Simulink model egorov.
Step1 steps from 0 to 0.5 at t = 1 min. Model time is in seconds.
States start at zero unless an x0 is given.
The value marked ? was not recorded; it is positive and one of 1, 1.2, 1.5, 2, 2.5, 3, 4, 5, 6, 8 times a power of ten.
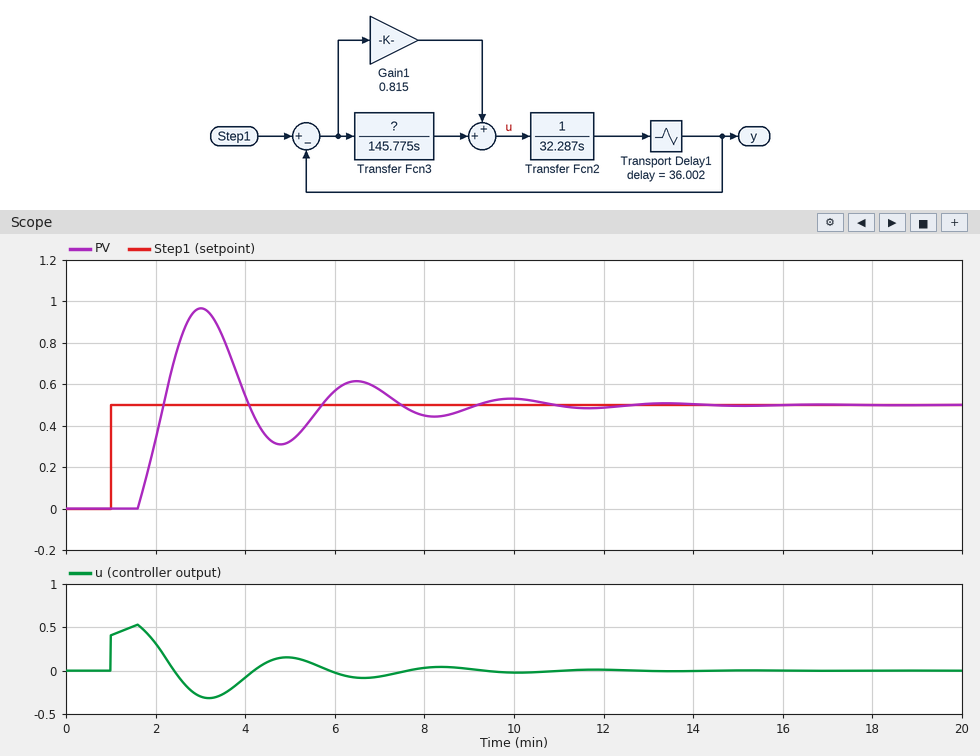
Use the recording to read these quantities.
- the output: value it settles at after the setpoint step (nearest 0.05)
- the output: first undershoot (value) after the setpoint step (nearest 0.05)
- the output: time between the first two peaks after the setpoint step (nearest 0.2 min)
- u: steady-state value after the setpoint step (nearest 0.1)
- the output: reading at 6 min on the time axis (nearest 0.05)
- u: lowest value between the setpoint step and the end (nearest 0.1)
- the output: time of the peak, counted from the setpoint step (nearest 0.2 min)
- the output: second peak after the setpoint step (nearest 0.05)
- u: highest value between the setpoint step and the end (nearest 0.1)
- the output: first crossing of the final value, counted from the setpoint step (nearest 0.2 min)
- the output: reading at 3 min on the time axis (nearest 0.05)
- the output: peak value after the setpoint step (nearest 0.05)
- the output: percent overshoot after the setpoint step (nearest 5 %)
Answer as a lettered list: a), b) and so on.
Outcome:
a) 0.50
b) 0.30
c) 3.4 min
d) 0.0
e) 0.55
f) -0.3
g) 2.0 min
h) 0.60
i) 0.5
j) 1.2 min
k) 0.95
l) 0.95
m) 95 %
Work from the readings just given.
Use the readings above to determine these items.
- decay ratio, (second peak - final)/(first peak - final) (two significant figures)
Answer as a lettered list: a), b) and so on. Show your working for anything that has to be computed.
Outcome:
a) (0.6 - 0.5) / (0.95 - 0.5) = 0.22
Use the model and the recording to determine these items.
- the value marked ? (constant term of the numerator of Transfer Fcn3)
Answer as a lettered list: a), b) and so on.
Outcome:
a) 1
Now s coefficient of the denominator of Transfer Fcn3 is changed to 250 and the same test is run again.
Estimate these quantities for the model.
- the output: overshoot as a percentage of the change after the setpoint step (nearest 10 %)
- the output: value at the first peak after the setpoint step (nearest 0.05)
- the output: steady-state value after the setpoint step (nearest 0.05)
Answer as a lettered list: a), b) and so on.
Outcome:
a) 70 %
b) 0.85
c) 0.50
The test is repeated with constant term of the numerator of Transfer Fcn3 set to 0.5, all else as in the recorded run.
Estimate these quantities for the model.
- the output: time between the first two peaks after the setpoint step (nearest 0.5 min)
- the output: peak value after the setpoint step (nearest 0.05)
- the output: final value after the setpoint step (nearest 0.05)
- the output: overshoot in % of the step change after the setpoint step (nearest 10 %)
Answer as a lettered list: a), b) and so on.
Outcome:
a) 3.0 min
b) 0.85
c) 0.50
d) 70 %
